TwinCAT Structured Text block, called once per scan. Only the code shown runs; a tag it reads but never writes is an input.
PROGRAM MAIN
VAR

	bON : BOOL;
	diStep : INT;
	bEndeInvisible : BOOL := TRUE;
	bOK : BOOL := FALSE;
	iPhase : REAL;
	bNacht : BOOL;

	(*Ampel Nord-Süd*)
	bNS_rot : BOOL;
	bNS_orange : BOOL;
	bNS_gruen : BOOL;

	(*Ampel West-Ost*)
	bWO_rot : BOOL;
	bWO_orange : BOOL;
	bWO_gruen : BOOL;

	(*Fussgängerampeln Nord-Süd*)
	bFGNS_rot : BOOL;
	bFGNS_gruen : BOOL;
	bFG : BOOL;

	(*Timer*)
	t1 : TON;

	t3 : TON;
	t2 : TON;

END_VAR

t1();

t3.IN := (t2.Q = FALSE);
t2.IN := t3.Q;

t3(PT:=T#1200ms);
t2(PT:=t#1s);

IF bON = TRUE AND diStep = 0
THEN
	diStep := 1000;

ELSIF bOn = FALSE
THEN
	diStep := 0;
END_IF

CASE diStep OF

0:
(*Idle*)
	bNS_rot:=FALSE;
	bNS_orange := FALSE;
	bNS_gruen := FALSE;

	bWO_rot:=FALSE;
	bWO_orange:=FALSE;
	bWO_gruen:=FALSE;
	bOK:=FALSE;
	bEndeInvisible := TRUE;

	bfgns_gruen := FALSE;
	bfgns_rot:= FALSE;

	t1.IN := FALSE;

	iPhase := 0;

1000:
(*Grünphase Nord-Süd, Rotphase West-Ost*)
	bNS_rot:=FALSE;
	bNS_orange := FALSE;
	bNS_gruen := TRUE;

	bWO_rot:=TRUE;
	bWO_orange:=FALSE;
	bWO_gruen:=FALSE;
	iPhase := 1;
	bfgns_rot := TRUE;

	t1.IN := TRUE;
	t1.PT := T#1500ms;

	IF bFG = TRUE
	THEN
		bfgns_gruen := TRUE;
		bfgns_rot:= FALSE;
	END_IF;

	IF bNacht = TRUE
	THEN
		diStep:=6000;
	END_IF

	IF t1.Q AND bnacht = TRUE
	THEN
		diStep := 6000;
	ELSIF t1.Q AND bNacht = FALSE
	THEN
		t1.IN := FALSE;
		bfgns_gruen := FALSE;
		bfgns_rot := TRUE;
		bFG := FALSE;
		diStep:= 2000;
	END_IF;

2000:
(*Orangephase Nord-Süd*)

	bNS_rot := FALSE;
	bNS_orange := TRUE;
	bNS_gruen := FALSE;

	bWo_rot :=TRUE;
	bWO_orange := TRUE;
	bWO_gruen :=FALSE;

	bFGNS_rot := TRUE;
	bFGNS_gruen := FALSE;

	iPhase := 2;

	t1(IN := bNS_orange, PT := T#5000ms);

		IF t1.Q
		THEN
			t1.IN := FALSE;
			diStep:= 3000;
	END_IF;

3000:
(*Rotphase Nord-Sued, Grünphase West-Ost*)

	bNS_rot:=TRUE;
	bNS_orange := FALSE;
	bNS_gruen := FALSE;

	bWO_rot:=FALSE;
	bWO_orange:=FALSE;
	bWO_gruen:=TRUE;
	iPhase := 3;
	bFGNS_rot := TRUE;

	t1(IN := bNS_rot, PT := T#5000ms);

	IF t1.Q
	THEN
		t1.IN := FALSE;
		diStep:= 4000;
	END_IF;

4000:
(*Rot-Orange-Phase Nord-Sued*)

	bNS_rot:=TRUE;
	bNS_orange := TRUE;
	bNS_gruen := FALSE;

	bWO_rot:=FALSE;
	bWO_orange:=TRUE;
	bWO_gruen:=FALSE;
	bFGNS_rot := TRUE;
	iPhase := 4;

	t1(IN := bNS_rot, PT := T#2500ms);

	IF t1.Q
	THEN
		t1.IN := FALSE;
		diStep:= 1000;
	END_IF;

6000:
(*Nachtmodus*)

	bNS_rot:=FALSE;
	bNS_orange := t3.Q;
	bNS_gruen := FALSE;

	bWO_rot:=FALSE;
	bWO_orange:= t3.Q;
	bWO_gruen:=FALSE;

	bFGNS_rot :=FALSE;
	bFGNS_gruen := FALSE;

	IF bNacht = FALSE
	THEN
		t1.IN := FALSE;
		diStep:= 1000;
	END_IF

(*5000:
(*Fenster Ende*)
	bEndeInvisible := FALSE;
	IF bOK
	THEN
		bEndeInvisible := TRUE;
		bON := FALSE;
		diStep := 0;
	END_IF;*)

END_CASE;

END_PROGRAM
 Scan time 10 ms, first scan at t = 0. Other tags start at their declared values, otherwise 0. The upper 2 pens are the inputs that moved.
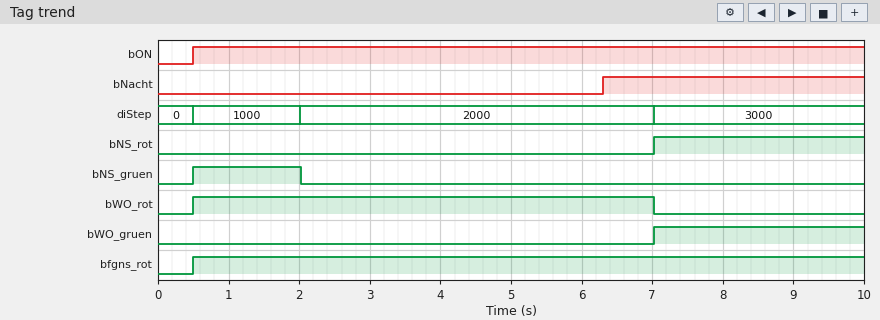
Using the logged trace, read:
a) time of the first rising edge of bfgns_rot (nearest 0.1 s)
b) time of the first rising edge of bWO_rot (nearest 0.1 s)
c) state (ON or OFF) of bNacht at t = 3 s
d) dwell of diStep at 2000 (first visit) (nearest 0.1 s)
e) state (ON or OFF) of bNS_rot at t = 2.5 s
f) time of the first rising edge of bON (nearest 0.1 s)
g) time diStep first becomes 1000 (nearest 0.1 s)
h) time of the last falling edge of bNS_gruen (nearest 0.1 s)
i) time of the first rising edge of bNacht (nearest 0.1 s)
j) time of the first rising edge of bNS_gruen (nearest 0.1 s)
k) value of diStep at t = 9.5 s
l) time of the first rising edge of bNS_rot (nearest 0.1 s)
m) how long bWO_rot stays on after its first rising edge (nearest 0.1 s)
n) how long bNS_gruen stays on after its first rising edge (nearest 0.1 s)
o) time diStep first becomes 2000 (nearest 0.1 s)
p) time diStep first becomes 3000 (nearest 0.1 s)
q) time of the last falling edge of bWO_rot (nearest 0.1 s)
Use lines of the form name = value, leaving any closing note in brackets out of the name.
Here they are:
time of the first rising edge of bfgns_rot = 0.5 s
time of the first rising edge of bWO_rot = 0.5 s
state (ON or OFF) of bNacht at t = 3 s = OFF
dwell of diStep at 2000 (first visit) = 5.0 s
state (ON or OFF) of bNS_rot at t = 2.5 s = OFF
time of the first rising edge of bON = 0.5 s
time diStep first becomes 1000 = 0.5 s
time of the last falling edge of bNS_gruen = 2.0 s
time of the first rising edge of bNacht = 6.3 s
time of the first rising edge of bNS_gruen = 0.5 s
value of diStep at t = 9.5 s = 3000
time of the first rising edge of bNS_rot = 7.0 s
how long bWO_rot stays on after its first rising edge = 6.5 s
how long bNS_gruen stays on after its first rising edge = 1.5 s
time diStep first becomes 2000 = 2.0 s
time diStep first becomes 3000 = 7.0 s
time of the last falling edge of bWO_rot = 7.0 s
